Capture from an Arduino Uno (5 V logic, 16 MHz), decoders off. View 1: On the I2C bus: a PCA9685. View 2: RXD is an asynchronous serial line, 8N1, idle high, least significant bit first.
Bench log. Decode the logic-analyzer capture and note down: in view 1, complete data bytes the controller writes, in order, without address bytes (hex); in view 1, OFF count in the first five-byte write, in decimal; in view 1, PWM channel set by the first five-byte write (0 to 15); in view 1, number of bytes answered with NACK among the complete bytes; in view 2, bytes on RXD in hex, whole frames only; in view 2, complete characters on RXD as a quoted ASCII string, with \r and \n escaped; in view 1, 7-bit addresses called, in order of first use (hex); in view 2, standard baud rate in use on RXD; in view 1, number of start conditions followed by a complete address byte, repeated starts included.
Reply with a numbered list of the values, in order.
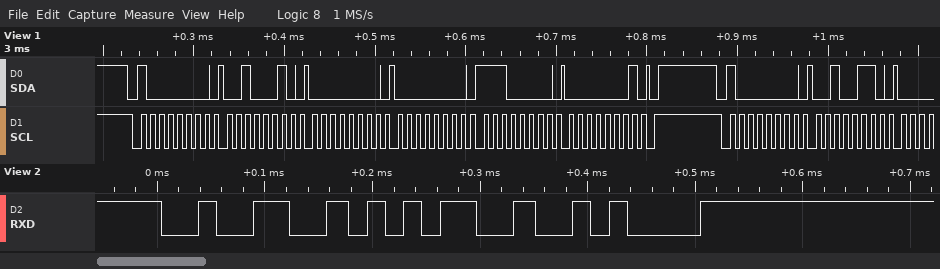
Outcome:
1. 22 00 00 E0 01 26
2. 480
3. 7
4. 0
5. 0x32 0x35 0x0A
6. "25\n"
7. 0x40
8. 57600 baud
9. 2
